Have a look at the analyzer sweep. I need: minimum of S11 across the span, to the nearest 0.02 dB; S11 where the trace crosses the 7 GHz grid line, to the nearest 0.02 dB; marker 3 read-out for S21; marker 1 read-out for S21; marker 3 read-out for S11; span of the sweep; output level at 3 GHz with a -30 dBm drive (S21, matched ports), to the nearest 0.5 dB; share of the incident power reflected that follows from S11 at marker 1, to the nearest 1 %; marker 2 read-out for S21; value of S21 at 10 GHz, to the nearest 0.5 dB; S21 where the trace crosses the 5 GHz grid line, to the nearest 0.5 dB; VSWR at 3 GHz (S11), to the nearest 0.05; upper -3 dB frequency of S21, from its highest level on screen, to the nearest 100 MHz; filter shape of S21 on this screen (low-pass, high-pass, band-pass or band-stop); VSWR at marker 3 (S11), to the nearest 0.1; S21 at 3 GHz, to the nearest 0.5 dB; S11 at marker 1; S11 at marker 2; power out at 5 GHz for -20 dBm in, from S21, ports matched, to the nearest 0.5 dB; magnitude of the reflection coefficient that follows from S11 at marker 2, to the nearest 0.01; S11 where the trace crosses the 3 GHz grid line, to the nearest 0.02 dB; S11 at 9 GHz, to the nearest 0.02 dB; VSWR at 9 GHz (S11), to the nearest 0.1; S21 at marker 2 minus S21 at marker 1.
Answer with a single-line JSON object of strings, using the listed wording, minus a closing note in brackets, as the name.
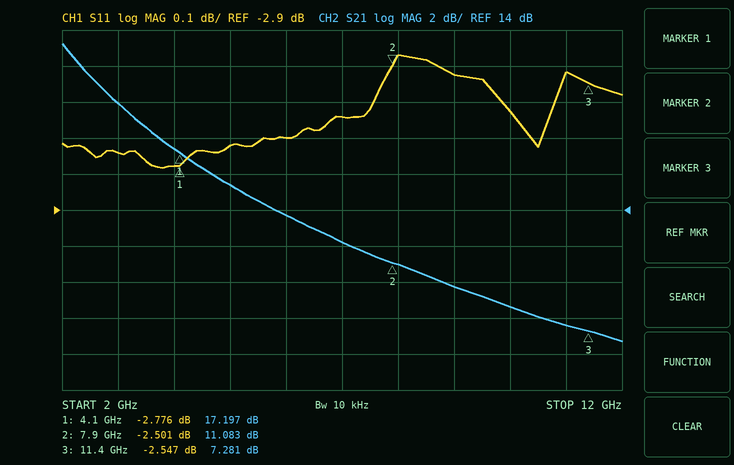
{"minimum of S11 across the span, to the nearest 0.02 dB": "-2.78 dB", "S11 where the trace crosses the 7 GHz grid line, to the nearest 0.02 dB": "-2.64 dB", "marker 3 read-out for S21": "7.281 dB", "marker 1 read-out for S21": "17.197 dB", "marker 3 read-out for S11": "-2.547 dB", "span of the sweep": "10 GHz", "output level at 3 GHz with a -30 dBm drive (S21, matched ports), to the nearest 0.5 dB": "-10.0 dBm", "share of the incident power reflected that follows from S11 at marker 1, to the nearest 1 %": "53 %", "marker 2 read-out for S21": "11.083 dB", "value of S21 at 10 GHz, to the nearest 0.5 dB": "8.5 dB", "S21 where the trace crosses the 5 GHz grid line, to the nearest 0.5 dB": "15.5 dB", "VSWR at 3 GHz (S11), to the nearest 0.05": "6.40", "upper -3 dB frequency of S21, from its highest level on screen, to the nearest 100 MHz": "2.9 GHz", "filter shape of S21 on this screen": "low-pass", "VSWR at marker 3 (S11), to the nearest 0.1": "6.9", "S21 at 3 GHz, to the nearest 0.5 dB": "20.0 dB", "S11 at marker 1": "-2.776 dB", "S11 at marker 2": "-2.501 dB", "power out at 5 GHz for -20 dBm in, from S21, ports matched, to the nearest 0.5 dB": "-4.5 dBm", "magnitude of the reflection coefficient that follows from S11 at marker 2, to the nearest 0.01": "0.75", "S11 where the trace crosses the 3 GHz grid line, to the nearest 0.02 dB": "-2.74 dB", "S11 at 9 GHz, to the nearest 0.02 dB": "-2.52 dB", "VSWR at 9 GHz (S11), to the nearest 0.1": "6.9", "S21 at marker 2 minus S21 at marker 1": "-6.114 dB"}
